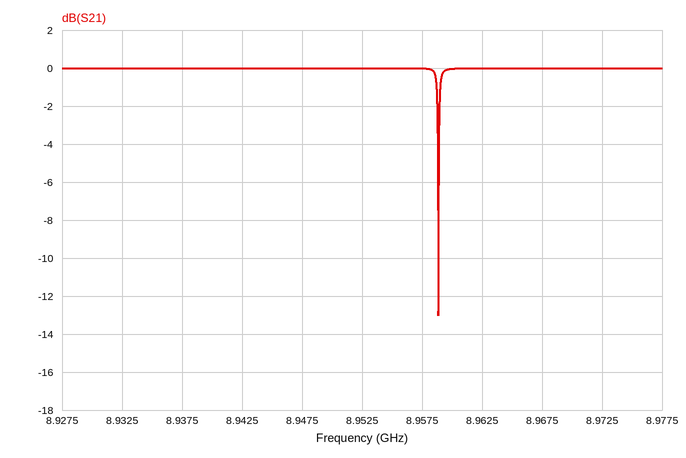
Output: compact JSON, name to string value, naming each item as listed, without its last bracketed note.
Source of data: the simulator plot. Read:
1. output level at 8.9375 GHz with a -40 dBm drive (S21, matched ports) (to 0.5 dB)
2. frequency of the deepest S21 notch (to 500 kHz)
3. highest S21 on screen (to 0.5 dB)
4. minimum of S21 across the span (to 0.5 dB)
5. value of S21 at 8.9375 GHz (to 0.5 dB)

{"output level at 8.9375 GHz with a -40 dBm drive (S21, matched ports)": "-40.0 dBm", "frequency of the deepest S21 notch": "8.9590 GHz", "highest S21 on screen": "0.0 dB", "minimum of S21 across the span": "-13.0 dB", "value of S21 at 8.9375 GHz": "0.0 dB"}
